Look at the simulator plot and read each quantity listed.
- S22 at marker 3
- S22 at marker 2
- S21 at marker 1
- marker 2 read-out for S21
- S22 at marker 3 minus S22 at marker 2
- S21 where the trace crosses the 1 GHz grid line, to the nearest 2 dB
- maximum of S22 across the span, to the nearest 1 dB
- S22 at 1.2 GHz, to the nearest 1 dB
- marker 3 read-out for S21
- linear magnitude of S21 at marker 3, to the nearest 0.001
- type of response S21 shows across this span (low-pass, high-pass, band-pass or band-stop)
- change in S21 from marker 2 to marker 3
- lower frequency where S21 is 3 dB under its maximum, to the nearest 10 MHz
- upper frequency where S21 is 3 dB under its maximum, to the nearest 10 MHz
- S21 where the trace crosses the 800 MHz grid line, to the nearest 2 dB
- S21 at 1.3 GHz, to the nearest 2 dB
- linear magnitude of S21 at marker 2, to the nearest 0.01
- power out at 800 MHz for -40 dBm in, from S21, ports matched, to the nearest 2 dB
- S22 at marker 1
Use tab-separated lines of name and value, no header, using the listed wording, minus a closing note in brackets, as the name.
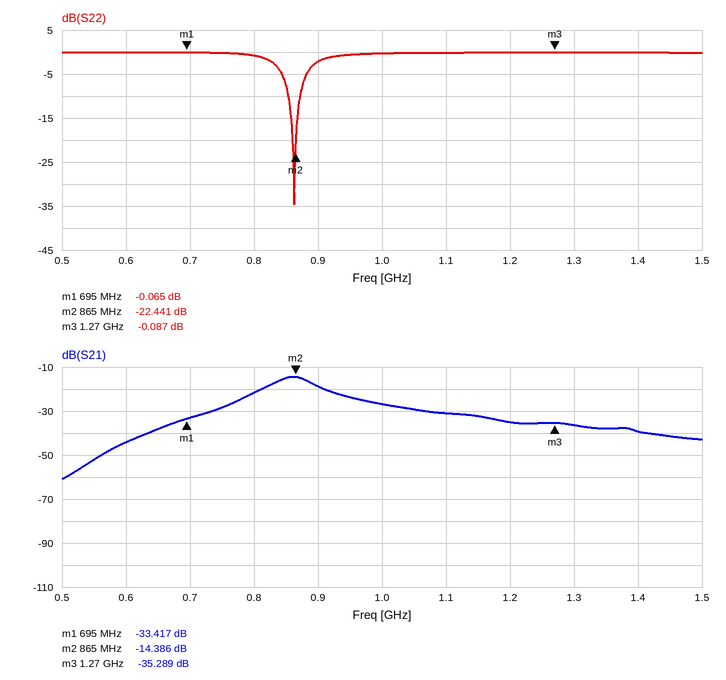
S22 at marker 3	-0.087 dB
S22 at marker 2	-22.441 dB
S21 at marker 1	-33.417 dB
marker 2 read-out for S21	-14.386 dB
S22 at marker 3 minus S22 at marker 2	22.354 dB
S21 where the trace crosses the 1 GHz grid line, to the nearest 2 dB	-26 dB
maximum of S22 across the span, to the nearest 1 dB	0 dB
S22 at 1.2 GHz, to the nearest 1 dB	0 dB
marker 3 read-out for S21	-35.289 dB
linear magnitude of S21 at marker 3, to the nearest 0.001	0.017
type of response S21 shows across this span	band-pass
change in S21 from marker 2 to marker 3	-20.903 dB
lower frequency where S21 is 3 dB under its maximum, to the nearest 10 MHz	830 MHz
upper frequency where S21 is 3 dB under its maximum, to the nearest 10 MHz	890 MHz
S21 where the trace crosses the 800 MHz grid line, to the nearest 2 dB	-22 dB
S21 at 1.3 GHz, to the nearest 2 dB	-36 dB
linear magnitude of S21 at marker 2, to the nearest 0.01	0.19
power out at 800 MHz for -40 dBm in, from S21, ports matched, to the nearest 2 dB	-62 dBm
S22 at marker 1	-0.065 dB
